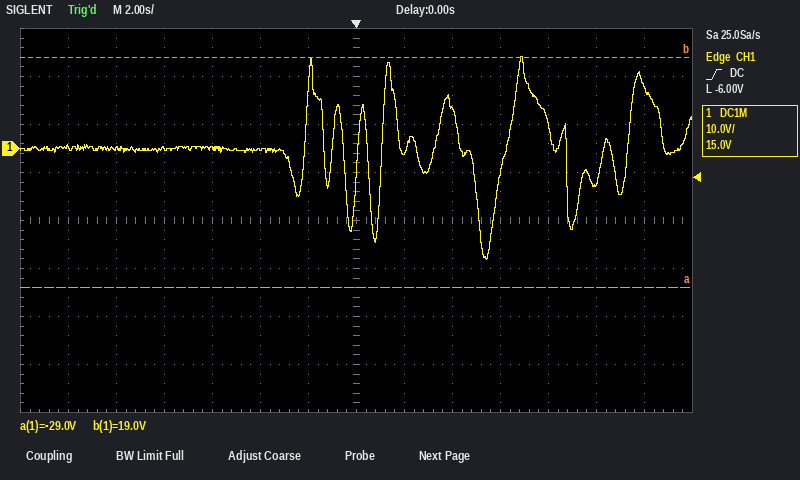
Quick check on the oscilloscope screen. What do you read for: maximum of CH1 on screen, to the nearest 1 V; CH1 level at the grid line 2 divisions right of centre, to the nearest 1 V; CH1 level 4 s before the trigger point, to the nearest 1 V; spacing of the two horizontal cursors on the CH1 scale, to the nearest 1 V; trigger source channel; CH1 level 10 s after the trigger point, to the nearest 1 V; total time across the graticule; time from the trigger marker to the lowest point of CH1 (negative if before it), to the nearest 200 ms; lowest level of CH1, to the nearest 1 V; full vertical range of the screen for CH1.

19 V
8 V
0 V
48 V
CH1
-7 V
28 s
+5.4 s
-23 V
80 V
